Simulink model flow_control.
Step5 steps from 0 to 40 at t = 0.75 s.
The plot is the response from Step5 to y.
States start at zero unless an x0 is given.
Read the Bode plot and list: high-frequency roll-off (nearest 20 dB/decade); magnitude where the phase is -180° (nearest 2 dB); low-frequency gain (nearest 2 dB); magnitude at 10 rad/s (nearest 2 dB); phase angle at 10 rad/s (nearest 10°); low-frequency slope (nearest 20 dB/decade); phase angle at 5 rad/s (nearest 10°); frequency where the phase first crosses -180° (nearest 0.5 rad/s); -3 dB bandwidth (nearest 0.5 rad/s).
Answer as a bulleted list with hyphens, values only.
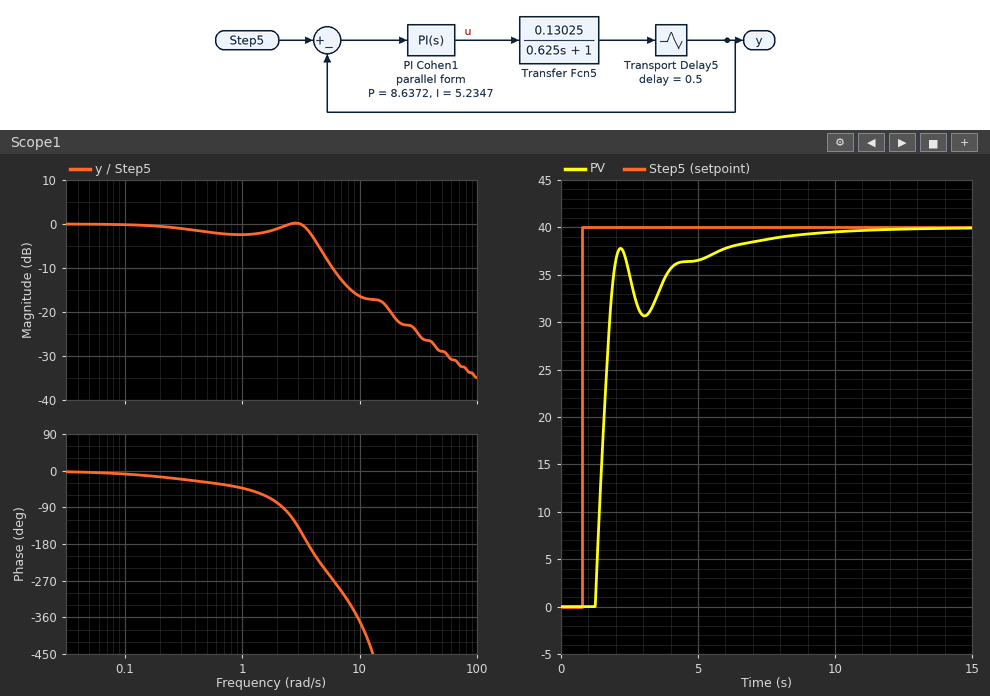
- -20 dB/decade
- -2 dB
- 0 dB
- -16 dB
- -370°
- 0 dB/decade
- -240°
- 3.5 rad/s
- 4.0 rad/s
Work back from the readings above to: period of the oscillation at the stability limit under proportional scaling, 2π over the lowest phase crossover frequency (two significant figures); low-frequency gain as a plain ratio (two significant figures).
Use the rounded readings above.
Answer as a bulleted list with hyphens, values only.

- 1.8 s
- 1.0
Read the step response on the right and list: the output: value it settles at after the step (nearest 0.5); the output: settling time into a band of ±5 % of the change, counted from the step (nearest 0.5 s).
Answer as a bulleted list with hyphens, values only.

- 40.0
- 5.5 s
